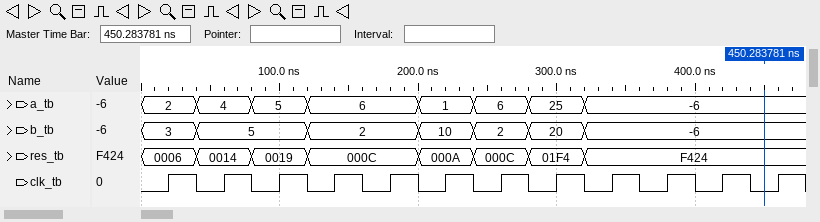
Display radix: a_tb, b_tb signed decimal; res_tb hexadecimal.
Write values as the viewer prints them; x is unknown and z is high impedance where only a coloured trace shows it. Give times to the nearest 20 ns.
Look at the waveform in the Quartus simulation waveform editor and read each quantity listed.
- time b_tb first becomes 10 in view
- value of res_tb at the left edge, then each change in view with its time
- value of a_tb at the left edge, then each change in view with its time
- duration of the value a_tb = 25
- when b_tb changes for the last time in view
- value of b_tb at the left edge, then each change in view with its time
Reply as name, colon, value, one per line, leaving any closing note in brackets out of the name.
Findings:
time b_tb first becomes 10 in view: 200 ns
value of res_tb at the left edge, then each change in view with its time: 0006, 0014 at 40 ns, 0019 at 80 ns, 000C at 120 ns, 000A at 200 ns, 000C at 240 ns, 01F4 at 280 ns, F424 at 320 ns
value of a_tb at the left edge, then each change in view with its time: 2, 4 at 40 ns, 5 at 80 ns, 6 at 120 ns, 1 at 200 ns, 6 at 240 ns, 25 at 280 ns, -6 at 320 ns
duration of the value a_tb = 25: 40 ns
when b_tb changes for the last time in view: 320 ns
value of b_tb at the left edge, then each change in view with its time: 3, 5 at 40 ns, 2 at 120 ns, 10 at 200 ns, 2 at 240 ns, 20 at 280 ns, -6 at 320 ns
